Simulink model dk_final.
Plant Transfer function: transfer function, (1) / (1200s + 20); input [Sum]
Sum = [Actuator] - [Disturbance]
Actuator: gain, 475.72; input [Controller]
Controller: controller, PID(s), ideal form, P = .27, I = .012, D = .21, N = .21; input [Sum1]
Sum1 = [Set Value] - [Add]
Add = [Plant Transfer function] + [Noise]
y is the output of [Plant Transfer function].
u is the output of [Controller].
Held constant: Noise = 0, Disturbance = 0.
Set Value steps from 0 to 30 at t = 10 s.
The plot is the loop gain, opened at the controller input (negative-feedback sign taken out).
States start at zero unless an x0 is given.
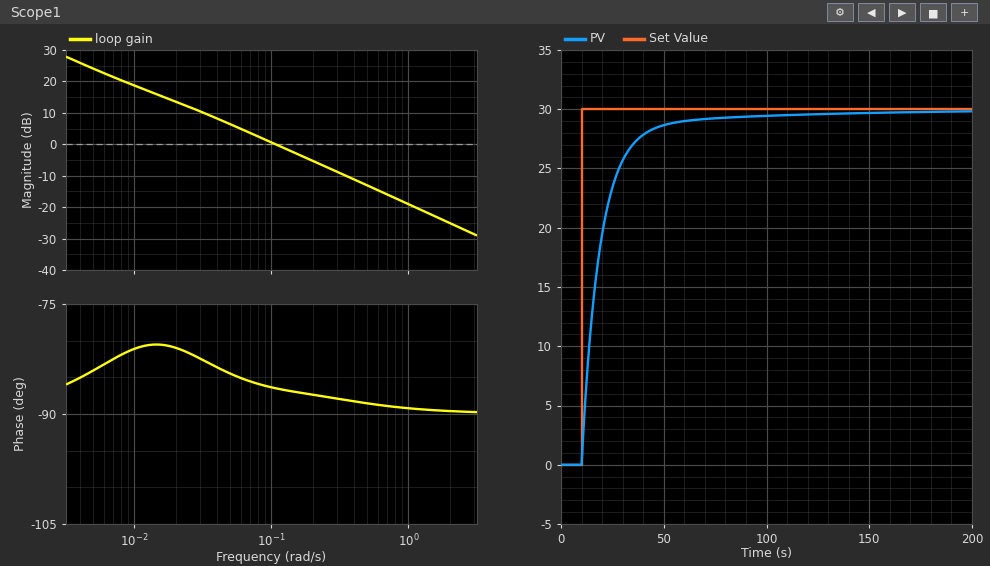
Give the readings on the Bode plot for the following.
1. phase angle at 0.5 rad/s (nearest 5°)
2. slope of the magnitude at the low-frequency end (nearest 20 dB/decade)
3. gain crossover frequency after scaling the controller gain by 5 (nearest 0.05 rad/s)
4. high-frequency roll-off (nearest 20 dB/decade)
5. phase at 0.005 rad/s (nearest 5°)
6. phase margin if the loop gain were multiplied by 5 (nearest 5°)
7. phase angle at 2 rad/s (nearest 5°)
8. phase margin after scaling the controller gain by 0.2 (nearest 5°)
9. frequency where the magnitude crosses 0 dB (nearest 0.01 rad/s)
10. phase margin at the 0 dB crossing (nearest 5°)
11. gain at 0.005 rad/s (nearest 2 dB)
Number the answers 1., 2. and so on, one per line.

1. -90°
2. -20 dB/decade
3. 0.55 rad/s
4. -20 dB/decade
5. -85°
6. 90°
7. -90°
8. 100°
9. 0.11 rad/s
10. 95°
11. 24 dB
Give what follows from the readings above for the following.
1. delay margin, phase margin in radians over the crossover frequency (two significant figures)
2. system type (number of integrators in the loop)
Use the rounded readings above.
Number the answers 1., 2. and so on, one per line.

1. 15 s
2. 1
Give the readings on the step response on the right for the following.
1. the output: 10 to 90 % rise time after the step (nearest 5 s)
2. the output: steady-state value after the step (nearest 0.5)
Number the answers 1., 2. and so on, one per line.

1. 25 s
2. 30.0
